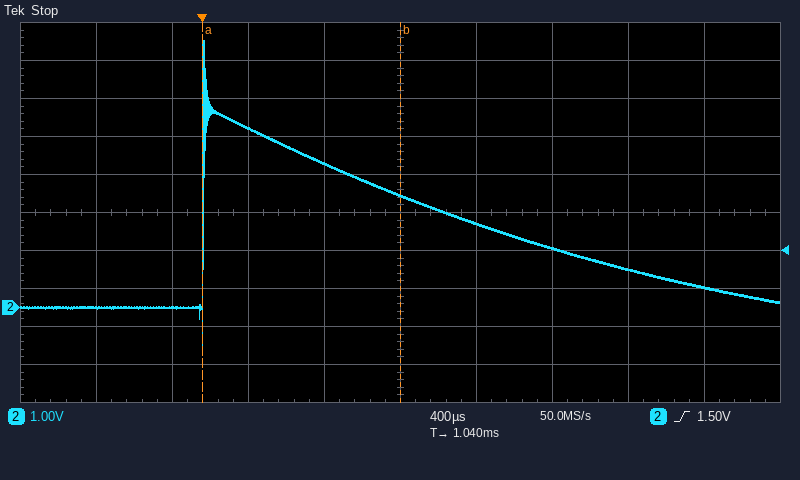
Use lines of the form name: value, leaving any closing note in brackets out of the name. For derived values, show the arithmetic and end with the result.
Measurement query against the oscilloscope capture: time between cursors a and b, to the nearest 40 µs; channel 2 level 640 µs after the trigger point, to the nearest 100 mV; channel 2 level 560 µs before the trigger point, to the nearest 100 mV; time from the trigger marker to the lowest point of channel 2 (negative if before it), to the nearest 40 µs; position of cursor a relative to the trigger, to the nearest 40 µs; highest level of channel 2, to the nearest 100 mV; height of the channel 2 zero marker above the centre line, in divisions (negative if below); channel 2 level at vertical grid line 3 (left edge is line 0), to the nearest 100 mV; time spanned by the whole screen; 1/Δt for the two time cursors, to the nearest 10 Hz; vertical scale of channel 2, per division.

time between cursors a and b, to the nearest 40 µs: 1.04 ms
channel 2 level 640 µs after the trigger point, to the nearest 100 mV: 3.8 V
channel 2 level 560 µs before the trigger point, to the nearest 100 mV: 0.0 V
time from the trigger marker to the lowest point of channel 2 (negative if before it), to the nearest 40 µs: 0 µs
position of cursor a relative to the trigger, to the nearest 40 µs: 0 µs
highest level of channel 2, to the nearest 100 mV: 7.0 V
height of the channel 2 zero marker above the centre line, in divisions: -2.5 div
channel 2 level at vertical grid line 3 (left edge is line 0), to the nearest 100 mV: 4.7 V
time spanned by the whole screen: 4 ms
1/Δt for the two time cursors, to the nearest 10 Hz: 1 / 1.04 ms ≈ 960 Hz
vertical scale of channel 2, per division: 1 V
